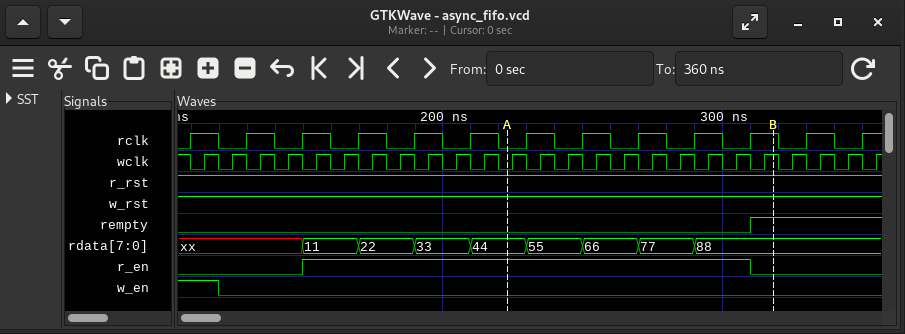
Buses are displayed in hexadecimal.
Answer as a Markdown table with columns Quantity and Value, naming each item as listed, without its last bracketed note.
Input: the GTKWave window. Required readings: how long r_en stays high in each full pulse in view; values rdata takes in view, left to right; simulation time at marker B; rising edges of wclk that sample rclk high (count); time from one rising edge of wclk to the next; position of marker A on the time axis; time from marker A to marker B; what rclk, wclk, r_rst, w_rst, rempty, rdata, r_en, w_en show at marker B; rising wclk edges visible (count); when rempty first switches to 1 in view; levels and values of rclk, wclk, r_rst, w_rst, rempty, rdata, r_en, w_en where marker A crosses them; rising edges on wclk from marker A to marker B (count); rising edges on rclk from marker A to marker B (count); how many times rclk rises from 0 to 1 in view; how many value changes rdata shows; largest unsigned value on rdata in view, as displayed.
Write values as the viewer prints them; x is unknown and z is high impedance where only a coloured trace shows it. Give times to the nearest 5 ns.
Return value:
| Quantity | Value |
|---|---|
| how long r_en stays high in each full pulse in view | 160 ns |
| values rdata takes in view, left to right | xx, 11, 22, 33, 44, 55, 66, 77, 88 |
| simulation time at marker B | 320 ns |
| rising edges of wclk that sample rclk high | 13 |
| time from one rising edge of wclk to the next | 10 ns |
| position of marker A on the time axis | 225 ns |
| time from marker A to marker B | 95 ns |
| what rclk, wclk, r_rst, w_rst, rempty, rdata, r_en, w_en show at marker B | rclk=1, wclk=1, r_rst=1, w_rst=1, rempty=1, rdata=88, r_en=0, w_en=0 |
| rising wclk edges visible | 25 |
| when rempty first switches to 1 in view | 310 ns |
| levels and values of rclk, wclk, r_rst, w_rst, rempty, rdata, r_en, w_en where marker A crosses them | rclk=0, wclk=0, r_rst=1, w_rst=1, rempty=0, rdata=44, r_en=1, w_en=0 |
| rising edges on wclk from marker A to marker B | 10 |
| rising edges on rclk from marker A to marker B | 5 |
| how many times rclk rises from 0 to 1 in view | 13 |
| how many value changes rdata shows | 8 |
| largest unsigned value on rdata in view, as displayed | 88 |
